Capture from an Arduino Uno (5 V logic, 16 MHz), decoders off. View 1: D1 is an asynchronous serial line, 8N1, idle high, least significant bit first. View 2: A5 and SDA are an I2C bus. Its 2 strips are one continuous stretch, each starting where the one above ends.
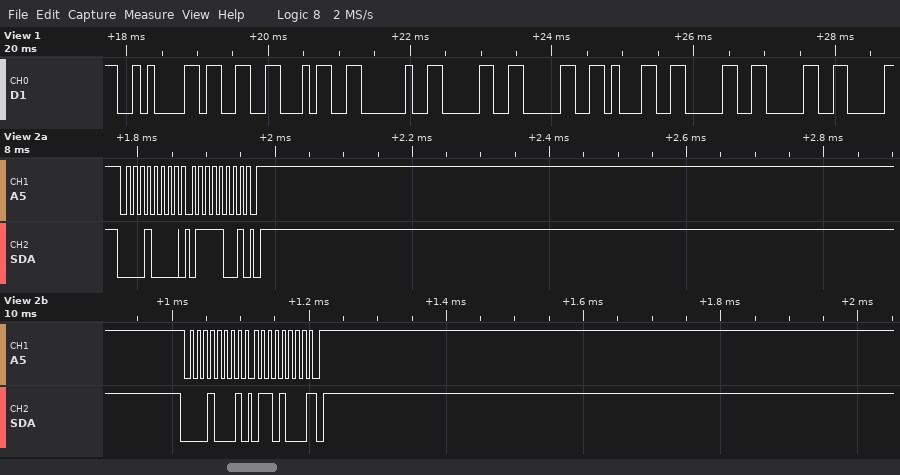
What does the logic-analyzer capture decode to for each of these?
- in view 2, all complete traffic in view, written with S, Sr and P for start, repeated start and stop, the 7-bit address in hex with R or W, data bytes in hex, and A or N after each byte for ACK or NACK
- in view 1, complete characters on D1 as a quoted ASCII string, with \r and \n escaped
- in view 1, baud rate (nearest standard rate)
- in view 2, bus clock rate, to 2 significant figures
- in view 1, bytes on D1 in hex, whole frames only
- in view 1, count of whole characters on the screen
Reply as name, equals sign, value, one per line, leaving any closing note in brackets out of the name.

in view 2, all complete traffic in view, written with S, Sr and P for start, repeated start and stop, the 7-bit address in hex with R or W, data bytes in hex, and A or N after each byte for ACK or NACK = S 08W A 79 A P S 08R A 68 N P
in view 1, complete characters on D1 as a quoted ASCII string, with \r and \n escaped = "\n34 00100"
in view 1, baud rate = 9600 baud
in view 2, bus clock rate, to 2 significant figures = 100 kHz
in view 1, bytes on D1 in hex, whole frames only = 0A 33 34 20 30 30 31 30 30
in view 1, count of whole characters on the screen = 9
